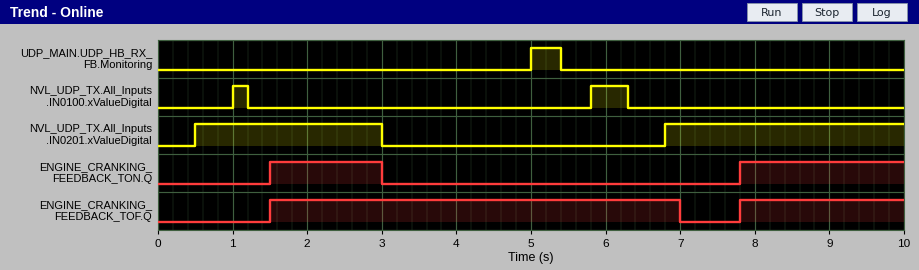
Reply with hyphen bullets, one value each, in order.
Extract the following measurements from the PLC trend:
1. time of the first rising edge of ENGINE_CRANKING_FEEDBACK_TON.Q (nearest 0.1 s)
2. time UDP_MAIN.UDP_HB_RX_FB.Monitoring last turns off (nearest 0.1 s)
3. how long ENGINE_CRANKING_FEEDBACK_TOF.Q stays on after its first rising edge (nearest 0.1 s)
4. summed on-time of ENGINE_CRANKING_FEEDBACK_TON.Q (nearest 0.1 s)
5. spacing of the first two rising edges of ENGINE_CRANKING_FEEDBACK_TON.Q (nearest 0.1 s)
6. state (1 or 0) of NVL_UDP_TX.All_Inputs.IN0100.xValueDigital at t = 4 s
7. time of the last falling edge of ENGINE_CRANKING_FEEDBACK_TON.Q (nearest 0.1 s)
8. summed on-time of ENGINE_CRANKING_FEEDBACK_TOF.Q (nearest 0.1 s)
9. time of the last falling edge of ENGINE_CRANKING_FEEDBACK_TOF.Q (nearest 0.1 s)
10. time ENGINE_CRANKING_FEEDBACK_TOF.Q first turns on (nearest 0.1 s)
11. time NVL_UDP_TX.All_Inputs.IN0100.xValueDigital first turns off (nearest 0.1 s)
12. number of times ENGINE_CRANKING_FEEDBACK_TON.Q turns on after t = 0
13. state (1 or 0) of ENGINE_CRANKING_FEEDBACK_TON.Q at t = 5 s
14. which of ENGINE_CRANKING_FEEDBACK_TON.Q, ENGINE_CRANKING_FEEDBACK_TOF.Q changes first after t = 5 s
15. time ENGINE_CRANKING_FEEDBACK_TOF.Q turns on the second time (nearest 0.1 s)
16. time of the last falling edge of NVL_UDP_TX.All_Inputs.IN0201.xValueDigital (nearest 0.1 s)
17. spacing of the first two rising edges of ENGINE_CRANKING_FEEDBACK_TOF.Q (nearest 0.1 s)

- 1.5 s
- 5.4 s
- 5.5 s
- 3.7 s
- 6.3 s
- 0
- 3.0 s
- 7.7 s
- 7.0 s
- 1.5 s
- 1.2 s
- 2
- 0
- ENGINE_CRANKING_FEEDBACK_TOF.Q
- 7.8 s
- 3.0 s
- 6.3 s
